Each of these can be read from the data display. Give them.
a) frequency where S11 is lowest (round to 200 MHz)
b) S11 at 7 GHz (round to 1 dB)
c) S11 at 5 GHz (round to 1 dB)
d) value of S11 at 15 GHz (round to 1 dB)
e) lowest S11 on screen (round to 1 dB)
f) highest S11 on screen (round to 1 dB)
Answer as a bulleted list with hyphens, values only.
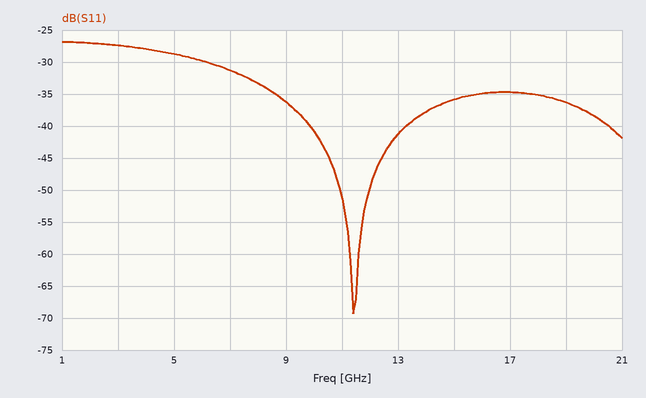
- 11.4 GHz
- -31 dB
- -29 dB
- -36 dB
- -69 dB
- -27 dB
